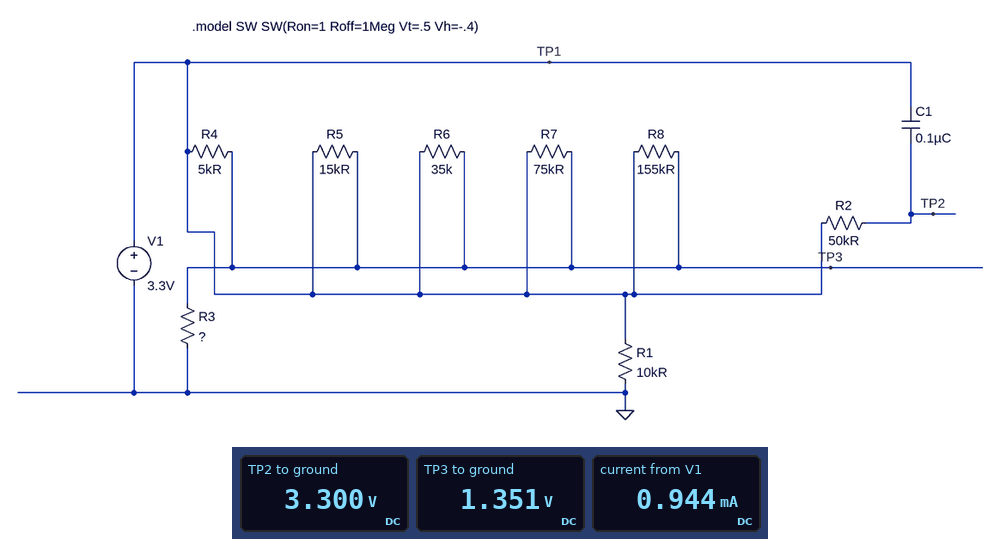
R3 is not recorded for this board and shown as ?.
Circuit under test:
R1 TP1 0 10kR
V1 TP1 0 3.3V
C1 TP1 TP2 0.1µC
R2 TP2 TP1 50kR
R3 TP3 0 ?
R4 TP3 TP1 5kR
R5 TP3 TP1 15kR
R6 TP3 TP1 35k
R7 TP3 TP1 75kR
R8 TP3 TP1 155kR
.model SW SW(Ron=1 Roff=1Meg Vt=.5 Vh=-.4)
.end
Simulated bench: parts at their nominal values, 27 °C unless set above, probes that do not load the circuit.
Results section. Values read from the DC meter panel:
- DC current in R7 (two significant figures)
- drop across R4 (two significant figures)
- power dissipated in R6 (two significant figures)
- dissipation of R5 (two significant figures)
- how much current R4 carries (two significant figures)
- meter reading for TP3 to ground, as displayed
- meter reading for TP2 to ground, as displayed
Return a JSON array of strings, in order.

["26 µA", "1.9 V", "110 µW", "250 µW", "390 µA", "1.351 V", "3.300 V"]
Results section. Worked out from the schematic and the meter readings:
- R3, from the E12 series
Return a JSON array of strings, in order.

["2.2 kΩ"]
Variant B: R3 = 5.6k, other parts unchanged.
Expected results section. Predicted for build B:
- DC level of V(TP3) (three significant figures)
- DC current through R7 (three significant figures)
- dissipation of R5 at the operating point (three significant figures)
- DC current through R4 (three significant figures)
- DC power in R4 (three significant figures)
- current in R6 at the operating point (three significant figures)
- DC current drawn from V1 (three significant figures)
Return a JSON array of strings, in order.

["2.11 V", "15.9 µA", "95.0 µW", "239 µA", "285 µW", "34.1 µA", "706 µA"]
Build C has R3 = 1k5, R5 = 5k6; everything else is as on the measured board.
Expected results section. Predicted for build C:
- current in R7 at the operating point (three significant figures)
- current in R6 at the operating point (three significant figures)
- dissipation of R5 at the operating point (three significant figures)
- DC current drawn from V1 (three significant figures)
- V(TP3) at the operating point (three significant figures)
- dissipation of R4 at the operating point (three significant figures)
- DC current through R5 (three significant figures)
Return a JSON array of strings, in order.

["26.8 µA", "57.5 µA", "723 µW", "1.19 mA", "1.29 V", "809 µW", "359 µA"]
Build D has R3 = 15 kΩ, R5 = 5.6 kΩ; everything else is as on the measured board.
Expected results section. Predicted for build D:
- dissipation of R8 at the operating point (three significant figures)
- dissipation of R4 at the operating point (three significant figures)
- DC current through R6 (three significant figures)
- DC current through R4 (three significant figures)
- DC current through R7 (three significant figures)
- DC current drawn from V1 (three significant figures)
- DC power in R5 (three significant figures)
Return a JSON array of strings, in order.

["1.28 µW", "39.7 µW", "12.7 µA", "89.1 µA", "5.94 µA", "520 µA", "35.5 µW"]
